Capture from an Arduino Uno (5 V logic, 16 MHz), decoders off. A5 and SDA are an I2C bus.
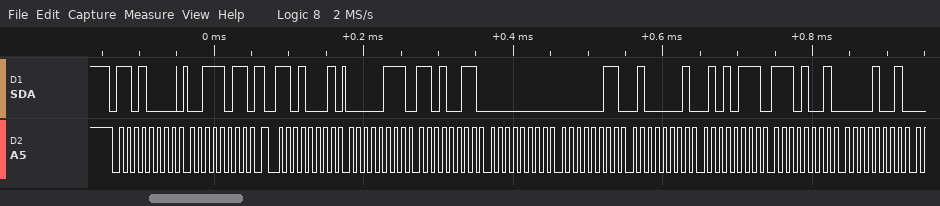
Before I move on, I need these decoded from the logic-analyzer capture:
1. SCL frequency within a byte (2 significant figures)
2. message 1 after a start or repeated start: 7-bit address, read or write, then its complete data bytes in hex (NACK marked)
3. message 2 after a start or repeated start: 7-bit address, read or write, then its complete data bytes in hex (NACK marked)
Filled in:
100 kHz
0x68 write: 3B
0x68 read: 07 D3 00 03 41 57 E9 09
